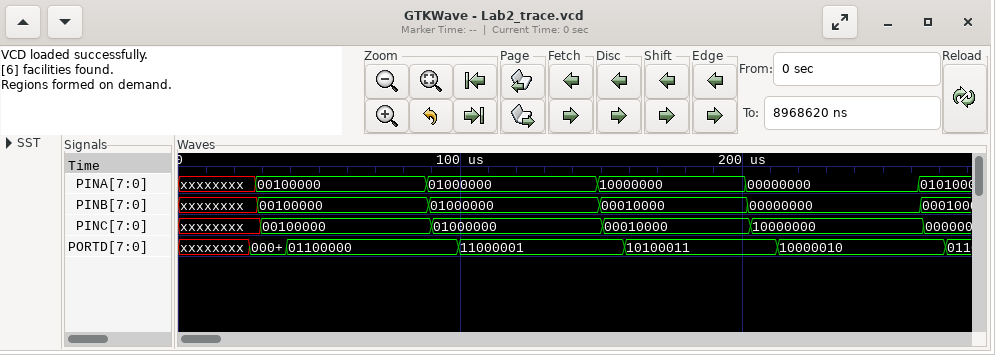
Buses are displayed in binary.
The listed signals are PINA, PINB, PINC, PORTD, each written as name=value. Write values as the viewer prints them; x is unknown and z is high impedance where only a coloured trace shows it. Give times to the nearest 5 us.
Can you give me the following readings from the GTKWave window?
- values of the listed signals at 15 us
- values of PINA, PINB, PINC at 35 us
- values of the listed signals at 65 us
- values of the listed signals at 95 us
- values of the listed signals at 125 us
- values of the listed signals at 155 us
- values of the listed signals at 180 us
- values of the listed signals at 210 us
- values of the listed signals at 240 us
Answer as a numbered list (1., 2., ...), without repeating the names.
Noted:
1. PINA=xxxxxxxx, PINB=xxxxxxxx, PINC=xxxxxxxx, PORTD=xxxxxxxx
2. PINA=00100000, PINB=00100000, PINC=00100000
3. PINA=00100000, PINB=00100000, PINC=00100000, PORTD=01100000
4. PINA=01000000, PINB=01000000, PINC=01000000, PORTD=01100000
5. PINA=01000000, PINB=01000000, PINC=01000000, PORTD=11000001
6. PINA=10000000, PINB=00010000, PINC=00010000, PORTD=11000001
7. PINA=10000000, PINB=00010000, PINC=00010000, PORTD=10100011
8. PINA=00000000, PINB=00000000, PINC=10000000, PORTD=10100011
9. PINA=00000000, PINB=00000000, PINC=10000000, PORTD=10000010
